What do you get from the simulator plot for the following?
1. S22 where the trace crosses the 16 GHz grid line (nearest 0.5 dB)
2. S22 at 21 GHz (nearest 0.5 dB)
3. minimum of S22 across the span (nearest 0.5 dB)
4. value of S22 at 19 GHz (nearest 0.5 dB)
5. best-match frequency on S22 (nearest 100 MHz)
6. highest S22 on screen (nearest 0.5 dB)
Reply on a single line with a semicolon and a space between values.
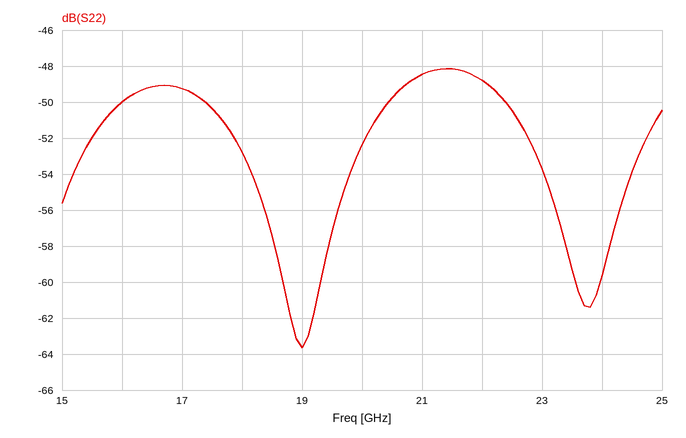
-50.0 dB; -48.5 dB; -63.5 dB; -63.5 dB; 19.0 GHz; -48.0 dB
